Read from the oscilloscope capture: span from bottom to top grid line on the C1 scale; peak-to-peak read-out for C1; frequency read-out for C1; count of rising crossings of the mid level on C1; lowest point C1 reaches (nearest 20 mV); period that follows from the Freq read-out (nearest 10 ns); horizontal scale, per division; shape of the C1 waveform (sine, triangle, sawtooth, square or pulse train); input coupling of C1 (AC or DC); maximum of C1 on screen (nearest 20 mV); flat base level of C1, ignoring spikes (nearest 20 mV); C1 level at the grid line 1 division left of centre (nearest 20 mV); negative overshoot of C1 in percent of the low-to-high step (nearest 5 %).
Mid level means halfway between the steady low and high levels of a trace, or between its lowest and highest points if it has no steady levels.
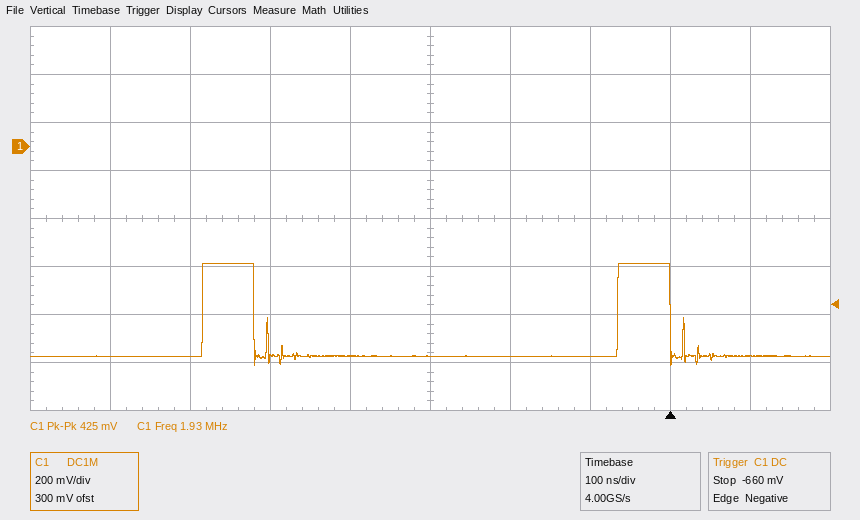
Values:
1.6 V
425 mV
1.93 MHz
2
-920 mV
520 ns
100 ns
pulse train
DC
-480 mV
-880 mV
-880 mV
10 %
